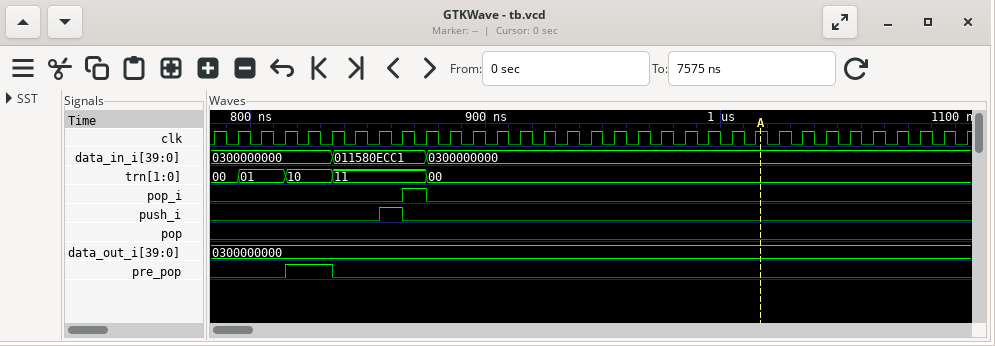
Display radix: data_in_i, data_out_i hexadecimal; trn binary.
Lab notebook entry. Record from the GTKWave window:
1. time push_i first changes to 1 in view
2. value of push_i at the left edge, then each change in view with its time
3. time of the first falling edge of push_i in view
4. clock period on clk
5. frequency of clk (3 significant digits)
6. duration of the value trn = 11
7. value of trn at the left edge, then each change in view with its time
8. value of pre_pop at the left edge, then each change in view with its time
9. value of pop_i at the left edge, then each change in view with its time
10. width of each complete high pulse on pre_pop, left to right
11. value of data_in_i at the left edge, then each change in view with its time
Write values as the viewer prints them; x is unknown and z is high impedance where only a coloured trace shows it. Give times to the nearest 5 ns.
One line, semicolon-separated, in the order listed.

855 ns; 0, 1 at 855 ns, 0 at 865 ns; 865 ns; 10 ns; 100 MHz; 40 ns; 00, 01 at 795 ns, 10 at 815 ns, 11 at 835 ns, 00 at 875 ns; 0, 1 at 815 ns, 0 at 835 ns; 0, 1 at 865 ns, 0 at 875 ns; 20 ns; 0300000000, 011580ECC1 at 835 ns, 0300000000 at 875 ns
